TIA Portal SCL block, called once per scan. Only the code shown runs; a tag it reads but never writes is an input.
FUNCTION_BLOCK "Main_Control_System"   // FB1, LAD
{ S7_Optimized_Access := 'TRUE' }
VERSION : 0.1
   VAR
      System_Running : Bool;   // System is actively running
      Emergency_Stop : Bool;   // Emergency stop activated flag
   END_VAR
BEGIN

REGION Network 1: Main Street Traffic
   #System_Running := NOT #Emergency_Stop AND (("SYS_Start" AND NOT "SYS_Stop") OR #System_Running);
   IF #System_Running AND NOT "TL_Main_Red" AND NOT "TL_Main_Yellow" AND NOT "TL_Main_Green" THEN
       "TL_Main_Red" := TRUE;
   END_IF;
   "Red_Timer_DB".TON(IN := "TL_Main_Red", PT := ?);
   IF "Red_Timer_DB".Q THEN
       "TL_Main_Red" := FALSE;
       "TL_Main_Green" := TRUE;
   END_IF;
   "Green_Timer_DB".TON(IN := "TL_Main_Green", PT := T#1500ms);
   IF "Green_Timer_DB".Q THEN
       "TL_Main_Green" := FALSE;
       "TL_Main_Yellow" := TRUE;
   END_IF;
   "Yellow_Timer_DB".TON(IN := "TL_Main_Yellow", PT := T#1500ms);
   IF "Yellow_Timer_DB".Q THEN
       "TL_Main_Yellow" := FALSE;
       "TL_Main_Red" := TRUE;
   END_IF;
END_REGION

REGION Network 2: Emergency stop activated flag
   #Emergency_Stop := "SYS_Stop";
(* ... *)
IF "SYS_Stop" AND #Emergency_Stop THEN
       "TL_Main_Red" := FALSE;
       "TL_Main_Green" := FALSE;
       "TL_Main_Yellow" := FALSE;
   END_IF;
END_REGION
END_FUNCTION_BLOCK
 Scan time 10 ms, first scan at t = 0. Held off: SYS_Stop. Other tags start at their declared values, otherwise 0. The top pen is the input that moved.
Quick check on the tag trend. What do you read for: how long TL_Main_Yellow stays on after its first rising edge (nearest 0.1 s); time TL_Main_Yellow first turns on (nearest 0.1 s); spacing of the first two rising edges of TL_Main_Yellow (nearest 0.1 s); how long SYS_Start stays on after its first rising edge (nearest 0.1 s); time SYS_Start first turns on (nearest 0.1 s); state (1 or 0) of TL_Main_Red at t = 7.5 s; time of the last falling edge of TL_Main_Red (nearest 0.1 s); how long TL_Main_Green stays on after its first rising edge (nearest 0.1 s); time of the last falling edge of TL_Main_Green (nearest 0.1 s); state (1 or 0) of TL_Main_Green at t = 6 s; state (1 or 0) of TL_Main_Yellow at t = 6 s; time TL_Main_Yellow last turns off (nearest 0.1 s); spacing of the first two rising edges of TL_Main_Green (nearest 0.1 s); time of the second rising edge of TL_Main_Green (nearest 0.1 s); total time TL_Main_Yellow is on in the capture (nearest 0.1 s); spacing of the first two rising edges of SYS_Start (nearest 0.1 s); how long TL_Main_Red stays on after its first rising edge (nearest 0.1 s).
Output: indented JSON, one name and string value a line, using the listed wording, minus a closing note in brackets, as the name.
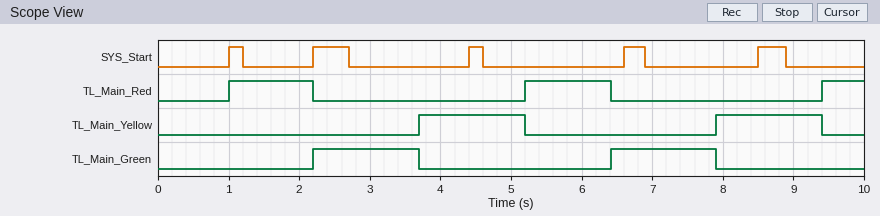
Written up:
{
  "how long TL_Main_Yellow stays on after its first rising edge": "1.5 s",
  "time TL_Main_Yellow first turns on": "3.7 s",
  "spacing of the first two rising edges of TL_Main_Yellow": "4.2 s",
  "how long SYS_Start stays on after its first rising edge": "0.2 s",
  "time SYS_Start first turns on": "1.0 s",
  "state (1 or 0) of TL_Main_Red at t = 7.5 s": "0",
  "time of the last falling edge of TL_Main_Red": "6.4 s",
  "how long TL_Main_Green stays on after its first rising edge": "1.5 s",
  "time of the last falling edge of TL_Main_Green": "7.9 s",
  "state (1 or 0) of TL_Main_Green at t = 6 s": "0",
  "state (1 or 0) of TL_Main_Yellow at t = 6 s": "0",
  "time TL_Main_Yellow last turns off": "9.4 s",
  "spacing of the first two rising edges of TL_Main_Green": "4.2 s",
  "time of the second rising edge of TL_Main_Green": "6.4 s",
  "total time TL_Main_Yellow is on in the capture": "3.0 s",
  "spacing of the first two rising edges of SYS_Start": "1.2 s",
  "how long TL_Main_Red stays on after its first rising edge": "1.2 s"
}
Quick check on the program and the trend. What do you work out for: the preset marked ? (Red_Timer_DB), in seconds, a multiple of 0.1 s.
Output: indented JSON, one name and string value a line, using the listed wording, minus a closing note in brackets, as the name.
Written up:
{
  "the preset marked ? (Red_Timer_DB), in seconds, a multiple of 0.1 s": "1.2 s"
}
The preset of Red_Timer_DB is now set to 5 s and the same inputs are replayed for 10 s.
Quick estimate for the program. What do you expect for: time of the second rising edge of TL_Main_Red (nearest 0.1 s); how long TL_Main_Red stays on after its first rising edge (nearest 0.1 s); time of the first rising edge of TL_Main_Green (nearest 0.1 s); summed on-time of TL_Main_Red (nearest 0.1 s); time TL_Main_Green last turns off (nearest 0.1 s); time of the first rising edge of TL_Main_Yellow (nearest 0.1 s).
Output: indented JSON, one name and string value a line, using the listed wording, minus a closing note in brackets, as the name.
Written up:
{
  "time of the second rising edge of TL_Main_Red": "9.0 s",
  "how long TL_Main_Red stays on after its first rising edge": "5.0 s",
  "time of the first rising edge of TL_Main_Green": "6.0 s",
  "summed on-time of TL_Main_Red": "6.0 s",
  "time TL_Main_Green last turns off": "7.5 s",
  "time of the first rising edge of TL_Main_Yellow": "7.5 s"
}
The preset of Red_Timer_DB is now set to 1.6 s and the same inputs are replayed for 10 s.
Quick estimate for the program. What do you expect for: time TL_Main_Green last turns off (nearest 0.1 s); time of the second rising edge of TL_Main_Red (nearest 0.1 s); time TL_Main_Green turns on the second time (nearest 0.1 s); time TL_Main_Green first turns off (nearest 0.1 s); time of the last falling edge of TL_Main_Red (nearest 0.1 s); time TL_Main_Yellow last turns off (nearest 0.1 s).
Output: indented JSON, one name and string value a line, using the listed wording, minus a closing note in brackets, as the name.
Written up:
{
  "time TL_Main_Green last turns off": "8.7 s",
  "time of the second rising edge of TL_Main_Red": "5.6 s",
  "time TL_Main_Green turns on the second time": "7.2 s",
  "time TL_Main_Green first turns off": "4.1 s",
  "time of the last falling edge of TL_Main_Red": "7.2 s",
  "time TL_Main_Yellow last turns off": "5.6 s"
}
